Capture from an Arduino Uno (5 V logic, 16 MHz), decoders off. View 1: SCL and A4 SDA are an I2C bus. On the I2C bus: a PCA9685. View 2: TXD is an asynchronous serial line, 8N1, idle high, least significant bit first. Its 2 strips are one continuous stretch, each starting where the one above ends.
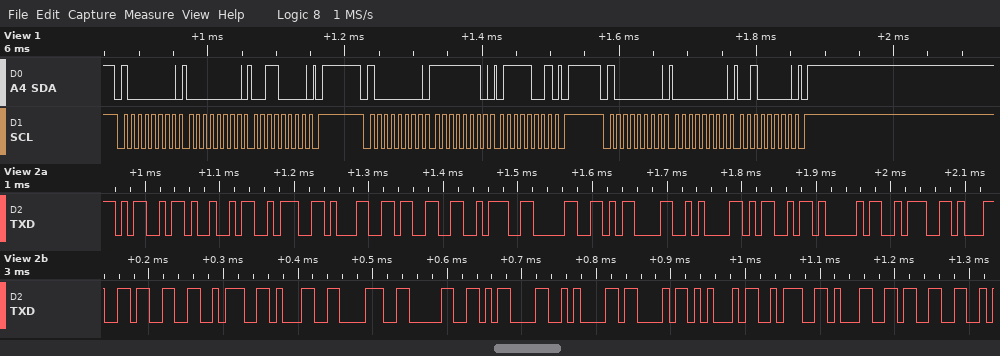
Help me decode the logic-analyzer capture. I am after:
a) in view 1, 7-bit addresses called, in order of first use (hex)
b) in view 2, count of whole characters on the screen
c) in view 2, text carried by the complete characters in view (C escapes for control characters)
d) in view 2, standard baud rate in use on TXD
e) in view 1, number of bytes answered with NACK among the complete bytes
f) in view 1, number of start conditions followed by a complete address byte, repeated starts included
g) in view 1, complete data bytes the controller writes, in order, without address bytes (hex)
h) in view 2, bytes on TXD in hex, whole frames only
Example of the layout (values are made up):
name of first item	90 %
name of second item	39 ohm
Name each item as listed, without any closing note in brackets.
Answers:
in view 1, 7-bit addresses called, in order of first use	0x40
in view 2, count of whole characters on the screen	25
in view 2, text carried by the complete characters in view	"MI:13:0\r\nMA:13:180\r\nCE:13"
in view 2, standard baud rate in use on TXD	115200 baud
in view 1, number of bytes answered with NACK among the complete bytes	0
in view 1, number of start conditions followed by a complete address byte, repeated starts included	3
in view 1, complete data bytes the controller writes, in order, without address bytes	00 30 FE 79 00 20
in view 2, bytes on TXD in hex, whole frames only	4D 49 3A 31 33 3A 30 0D 0A 4D 41 3A 31 33 3A 31 38 30 0D 0A 43 45 3A 31 33
